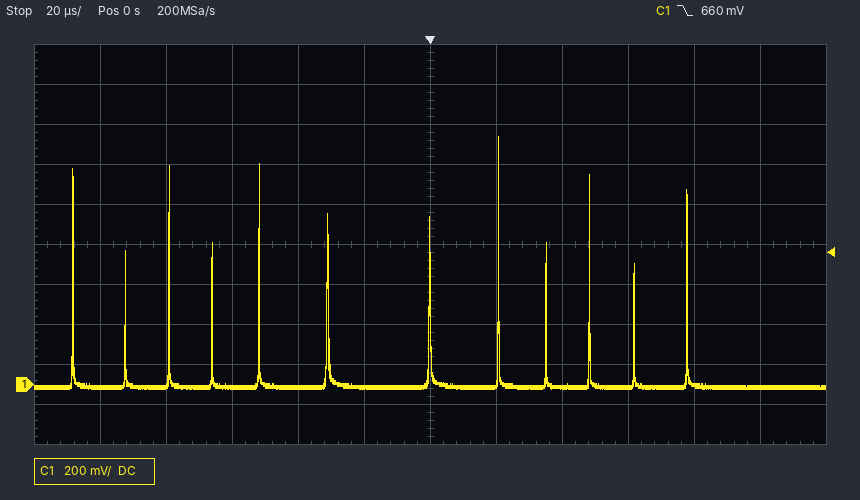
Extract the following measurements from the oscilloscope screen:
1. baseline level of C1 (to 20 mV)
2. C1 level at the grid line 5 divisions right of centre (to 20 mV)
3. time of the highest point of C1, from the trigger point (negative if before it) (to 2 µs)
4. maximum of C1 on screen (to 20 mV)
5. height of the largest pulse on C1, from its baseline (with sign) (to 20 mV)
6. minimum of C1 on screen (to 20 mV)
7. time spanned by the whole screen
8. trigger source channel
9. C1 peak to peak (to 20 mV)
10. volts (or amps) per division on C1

-20 mV
-20 mV
+20 µs
1.24 V
+1.26 V
-20 mV
240 µs
C1
1.26 V
200 mV
